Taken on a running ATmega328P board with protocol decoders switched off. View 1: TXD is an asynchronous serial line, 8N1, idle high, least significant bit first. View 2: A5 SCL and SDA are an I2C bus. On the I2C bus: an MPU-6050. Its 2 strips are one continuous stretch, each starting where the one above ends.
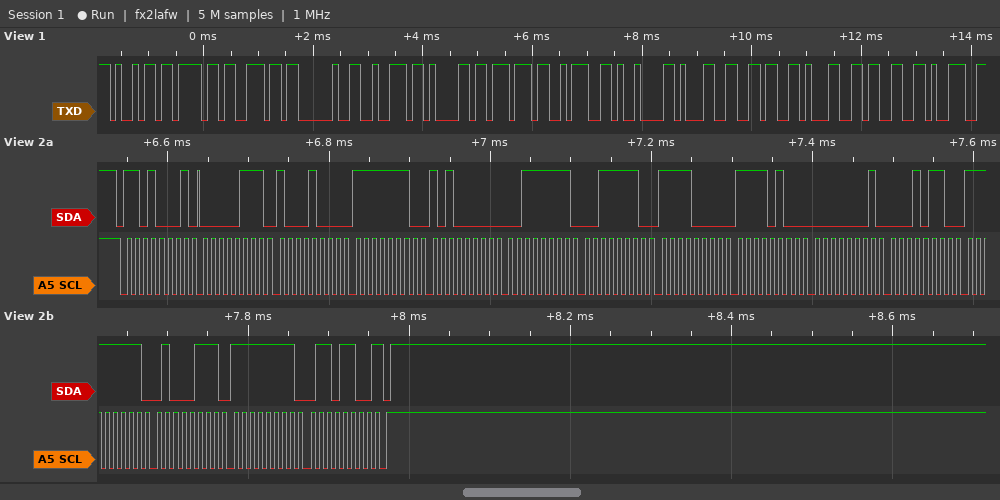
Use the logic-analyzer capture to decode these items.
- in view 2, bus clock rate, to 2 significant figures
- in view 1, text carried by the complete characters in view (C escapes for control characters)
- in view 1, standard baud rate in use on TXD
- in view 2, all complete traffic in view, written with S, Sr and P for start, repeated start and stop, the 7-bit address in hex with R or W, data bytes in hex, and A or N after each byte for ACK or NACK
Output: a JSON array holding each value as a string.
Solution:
["100 kHz", "\"ion raw:\\t16139\"", "9600 baud", "S 68R A 07 A 88 A FE A A0 A 3F A 3E A F0 A F4 A 01 A 16 A FF A 47 A FF A 6C N P"]
